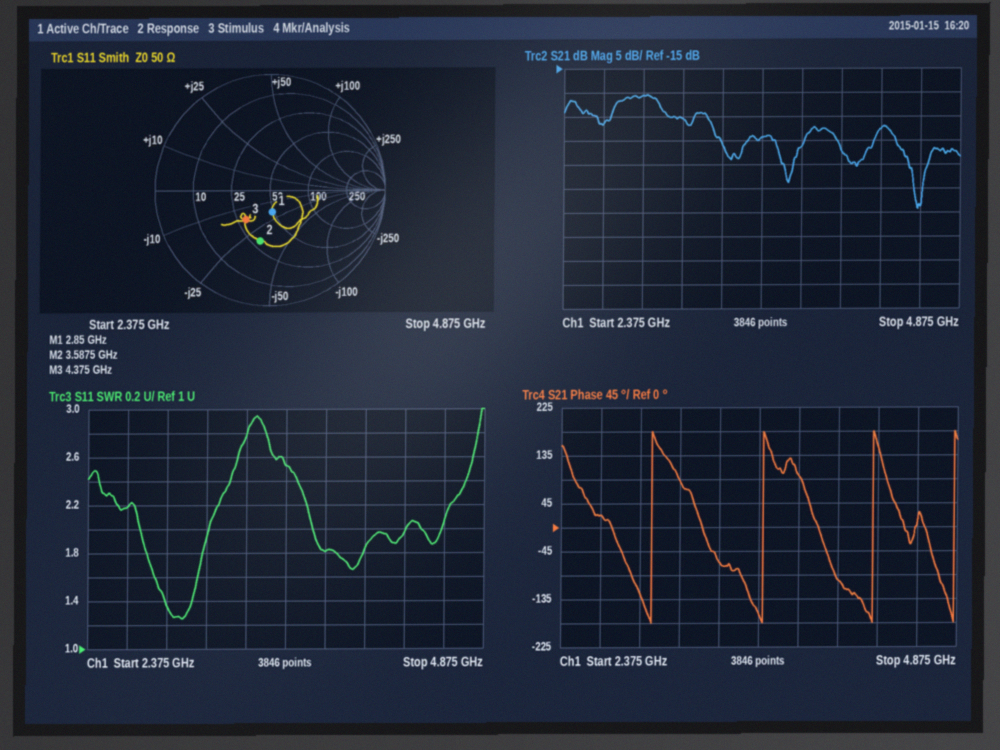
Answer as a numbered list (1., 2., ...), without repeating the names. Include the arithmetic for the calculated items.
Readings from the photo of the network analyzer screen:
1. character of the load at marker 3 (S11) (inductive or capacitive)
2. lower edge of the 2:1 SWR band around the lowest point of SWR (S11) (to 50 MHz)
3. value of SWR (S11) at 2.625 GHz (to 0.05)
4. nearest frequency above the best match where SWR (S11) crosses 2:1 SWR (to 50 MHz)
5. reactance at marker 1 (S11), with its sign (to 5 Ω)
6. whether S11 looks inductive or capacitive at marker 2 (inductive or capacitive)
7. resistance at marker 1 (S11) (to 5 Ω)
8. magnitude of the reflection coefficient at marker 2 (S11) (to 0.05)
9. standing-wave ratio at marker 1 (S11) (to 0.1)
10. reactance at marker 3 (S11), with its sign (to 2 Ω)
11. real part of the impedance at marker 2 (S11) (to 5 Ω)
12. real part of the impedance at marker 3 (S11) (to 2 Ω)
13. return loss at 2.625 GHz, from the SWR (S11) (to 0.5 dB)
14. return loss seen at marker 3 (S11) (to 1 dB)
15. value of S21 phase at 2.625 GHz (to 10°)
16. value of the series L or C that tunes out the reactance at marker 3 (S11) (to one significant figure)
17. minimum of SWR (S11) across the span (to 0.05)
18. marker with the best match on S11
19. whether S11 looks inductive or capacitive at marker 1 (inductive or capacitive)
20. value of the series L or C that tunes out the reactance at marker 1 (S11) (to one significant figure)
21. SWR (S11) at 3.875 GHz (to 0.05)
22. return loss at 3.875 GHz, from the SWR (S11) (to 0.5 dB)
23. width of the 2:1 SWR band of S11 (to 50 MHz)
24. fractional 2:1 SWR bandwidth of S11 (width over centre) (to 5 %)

1. capacitive
2. 2.70 GHz
3. 2.20
4. 3.15 GHz
5. -20 Ω
6. capacitive
7. 50 Ω
8. 0.45
9. 1.5
10. -16 Ω
11. 30 Ω
12. 30 Ω
13. −20 log10((2.2 − 1)/(2.2 + 1)) ≈ 8.5 dB
14. 10 dB
15. 20°
16. L = 16 Ω/(2π × 4.375 GHz) ≈ 582 pH, so 600 pH to one significant figure
17. 1.25
18. marker 1
19. capacitive
20. L = 20 Ω/(2π × 2.85 GHz) ≈ 1 nH
21. 1.80
22. −20 log10((1.8 − 1)/(1.8 + 1)) ≈ 10.9 dB, so 11.0 dB to the nearest 0.5 dB
23. 3.15 GHz − 2.70 GHz = 450 MHz
24. 450 MHz / 2.925 GHz ≈ 15 %
